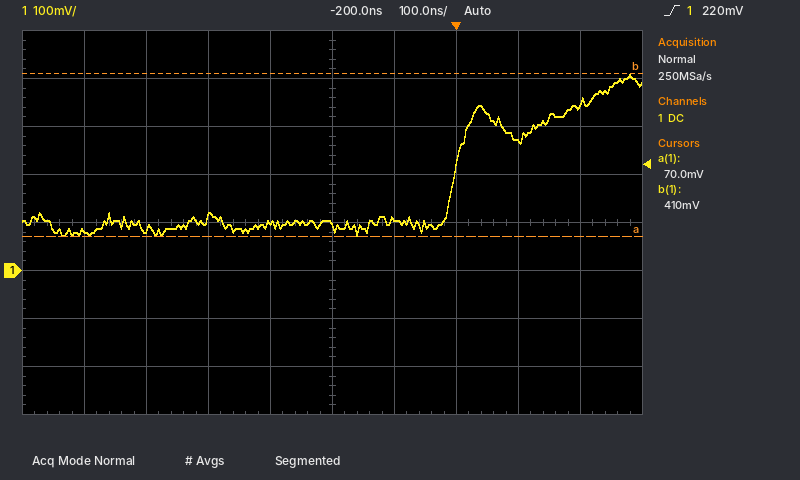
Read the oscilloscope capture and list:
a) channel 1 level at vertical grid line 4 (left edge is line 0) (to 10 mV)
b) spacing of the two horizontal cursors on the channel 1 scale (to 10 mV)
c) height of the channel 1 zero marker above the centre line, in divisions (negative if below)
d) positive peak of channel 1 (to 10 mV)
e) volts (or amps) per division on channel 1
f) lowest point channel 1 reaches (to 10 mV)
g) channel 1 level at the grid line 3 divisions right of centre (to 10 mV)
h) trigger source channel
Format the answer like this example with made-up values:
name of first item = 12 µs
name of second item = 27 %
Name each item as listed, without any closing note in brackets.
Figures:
channel 1 level at vertical grid line 4 (left edge is line 0) = 100 mV
spacing of the two horizontal cursors on the channel 1 scale = 340 mV
height of the channel 1 zero marker above the centre line, in divisions = -1.0 div
positive peak of channel 1 = 410 mV
volts (or amps) per division on channel 1 = 100 mV
lowest point channel 1 reaches = 70 mV
channel 1 level at the grid line 3 divisions right of centre = 270 mV
trigger source channel = channel 1
